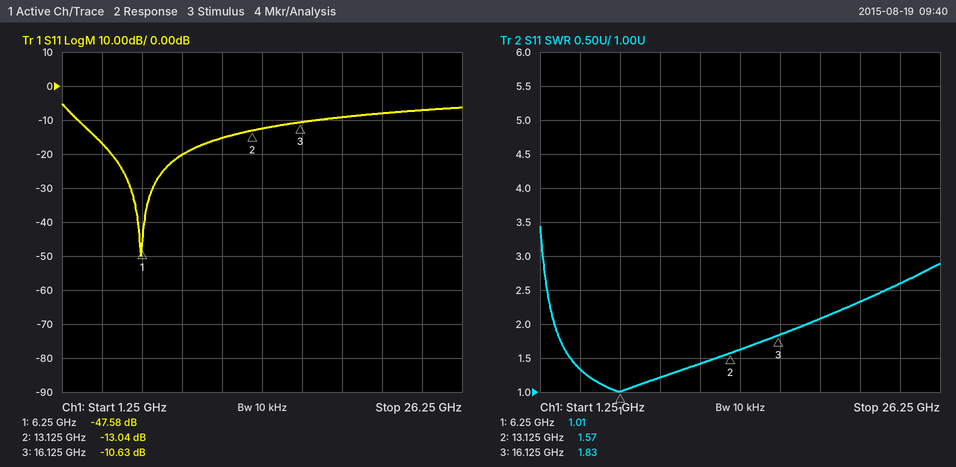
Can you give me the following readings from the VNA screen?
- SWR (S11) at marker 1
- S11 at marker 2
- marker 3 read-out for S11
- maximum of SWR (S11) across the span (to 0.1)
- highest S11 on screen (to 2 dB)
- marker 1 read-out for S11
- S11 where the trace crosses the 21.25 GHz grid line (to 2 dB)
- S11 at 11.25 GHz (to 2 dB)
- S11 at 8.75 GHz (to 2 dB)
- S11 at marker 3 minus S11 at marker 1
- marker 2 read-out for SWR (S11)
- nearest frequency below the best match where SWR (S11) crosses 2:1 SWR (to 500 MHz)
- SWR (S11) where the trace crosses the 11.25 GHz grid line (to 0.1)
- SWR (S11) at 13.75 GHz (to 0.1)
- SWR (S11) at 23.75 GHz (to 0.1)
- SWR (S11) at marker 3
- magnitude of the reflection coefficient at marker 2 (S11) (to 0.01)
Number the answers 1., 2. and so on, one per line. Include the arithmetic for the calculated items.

1. 1.01
2. -13.04 dB
3. -10.63 dB
4. 3.4
5. -6 dB
6. -47.58 dB
7. -8 dB
8. -16 dB
9. -20 dB
10. -10.63 − (-47.58) = 36.95 dB
11. 1.57
12. 2.0 GHz
13. 1.4
14. 1.6
15. 2.6
16. 1.83
17. 10^(-13.04/20) ≈ 0.22
